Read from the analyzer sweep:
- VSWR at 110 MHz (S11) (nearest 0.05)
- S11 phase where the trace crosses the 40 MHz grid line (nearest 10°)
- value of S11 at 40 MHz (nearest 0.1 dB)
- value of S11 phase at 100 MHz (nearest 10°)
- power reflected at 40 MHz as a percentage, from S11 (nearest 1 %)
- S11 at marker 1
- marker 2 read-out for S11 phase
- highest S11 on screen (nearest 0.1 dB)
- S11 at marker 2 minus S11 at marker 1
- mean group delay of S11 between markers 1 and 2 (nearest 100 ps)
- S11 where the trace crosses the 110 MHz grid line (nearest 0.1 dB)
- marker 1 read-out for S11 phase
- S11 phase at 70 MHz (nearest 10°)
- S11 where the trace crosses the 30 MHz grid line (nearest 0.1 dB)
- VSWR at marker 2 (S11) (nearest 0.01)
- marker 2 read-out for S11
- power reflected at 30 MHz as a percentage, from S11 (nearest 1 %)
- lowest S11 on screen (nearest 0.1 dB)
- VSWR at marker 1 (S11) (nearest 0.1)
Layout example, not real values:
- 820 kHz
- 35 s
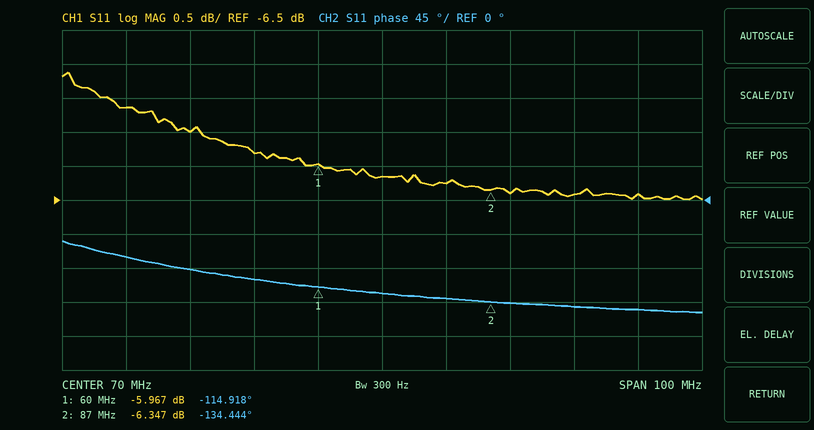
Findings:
- 2.85
- -90°
- -5.5 dB
- -140°
- 28 %
- -5.967 dB
- -134.444°
- -4.6 dB
- -0.380 dB
- 2.0 ns
- -6.4 dB
- -114.918°
- -120°
- -5.1 dB
- 2.86
- -6.347 dB
- 31 %
- -6.5 dB
- 3.0
